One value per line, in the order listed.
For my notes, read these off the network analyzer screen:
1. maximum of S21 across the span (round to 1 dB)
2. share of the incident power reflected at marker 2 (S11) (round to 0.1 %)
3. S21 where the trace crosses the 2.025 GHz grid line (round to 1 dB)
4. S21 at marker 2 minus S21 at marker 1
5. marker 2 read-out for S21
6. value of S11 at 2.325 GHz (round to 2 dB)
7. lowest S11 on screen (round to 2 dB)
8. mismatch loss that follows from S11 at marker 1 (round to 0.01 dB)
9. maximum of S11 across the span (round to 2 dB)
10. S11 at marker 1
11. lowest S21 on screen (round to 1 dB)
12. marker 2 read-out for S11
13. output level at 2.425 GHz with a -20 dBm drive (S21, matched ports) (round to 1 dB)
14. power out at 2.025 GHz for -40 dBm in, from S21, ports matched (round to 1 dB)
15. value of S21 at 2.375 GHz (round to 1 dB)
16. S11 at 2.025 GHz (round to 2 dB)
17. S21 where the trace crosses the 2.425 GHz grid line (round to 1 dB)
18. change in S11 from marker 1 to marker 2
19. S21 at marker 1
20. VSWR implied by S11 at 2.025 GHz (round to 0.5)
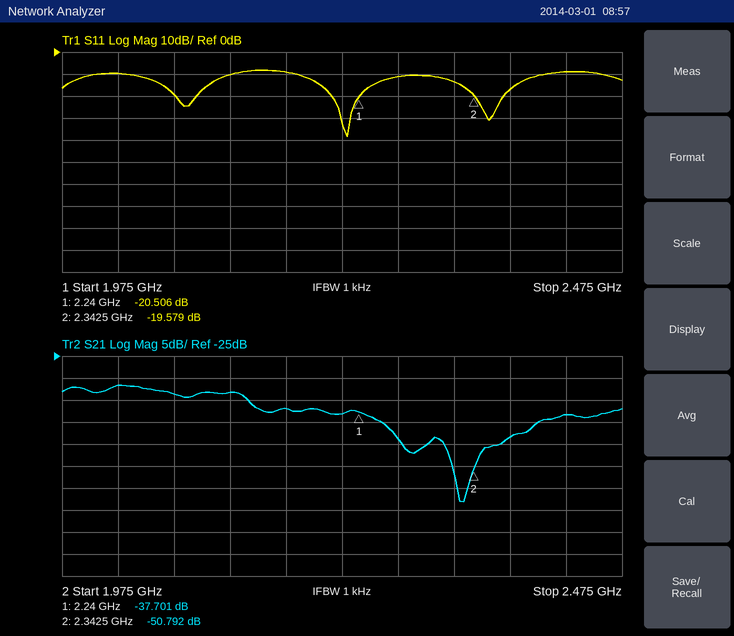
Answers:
-32 dB
1.1 %
-32 dB
-13.091 dB
-50.792 dB
-14 dB
-38 dB
0.04 dB
-8 dB
-20.506 dB
-58 dB
-19.579 dB
-58 dBm
-72 dBm
-43 dB
-10 dB
-38 dB
0.927 dB
-37.701 dB
2.0
